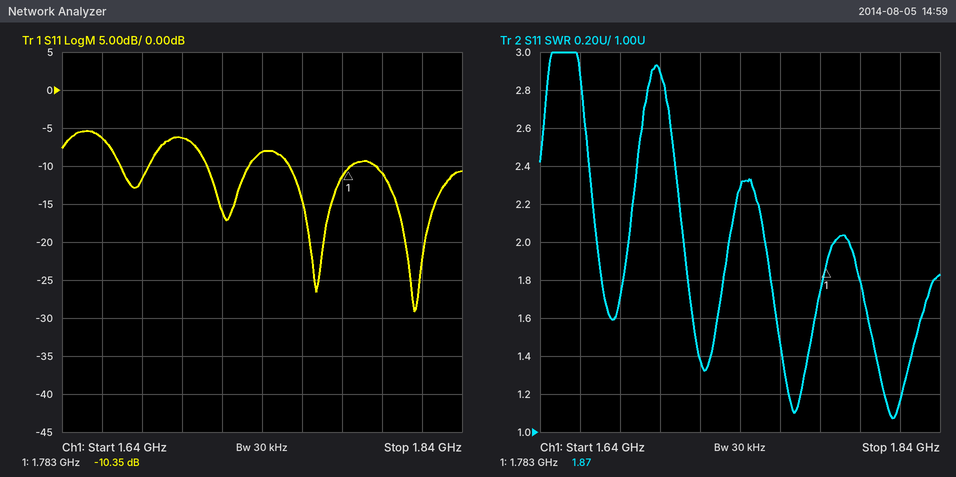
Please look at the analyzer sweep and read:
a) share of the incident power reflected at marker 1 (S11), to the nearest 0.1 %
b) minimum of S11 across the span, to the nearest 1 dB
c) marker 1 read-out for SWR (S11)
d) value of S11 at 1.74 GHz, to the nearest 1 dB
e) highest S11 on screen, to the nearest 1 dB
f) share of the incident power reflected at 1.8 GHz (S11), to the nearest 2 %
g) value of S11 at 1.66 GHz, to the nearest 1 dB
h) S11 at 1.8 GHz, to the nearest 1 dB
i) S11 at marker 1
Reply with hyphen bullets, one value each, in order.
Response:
- 9.2 %
- -29 dB
- 1.87
- -8 dB
- -5 dB
- 8 %
- -6 dB
- -11 dB
- -10.35 dB
